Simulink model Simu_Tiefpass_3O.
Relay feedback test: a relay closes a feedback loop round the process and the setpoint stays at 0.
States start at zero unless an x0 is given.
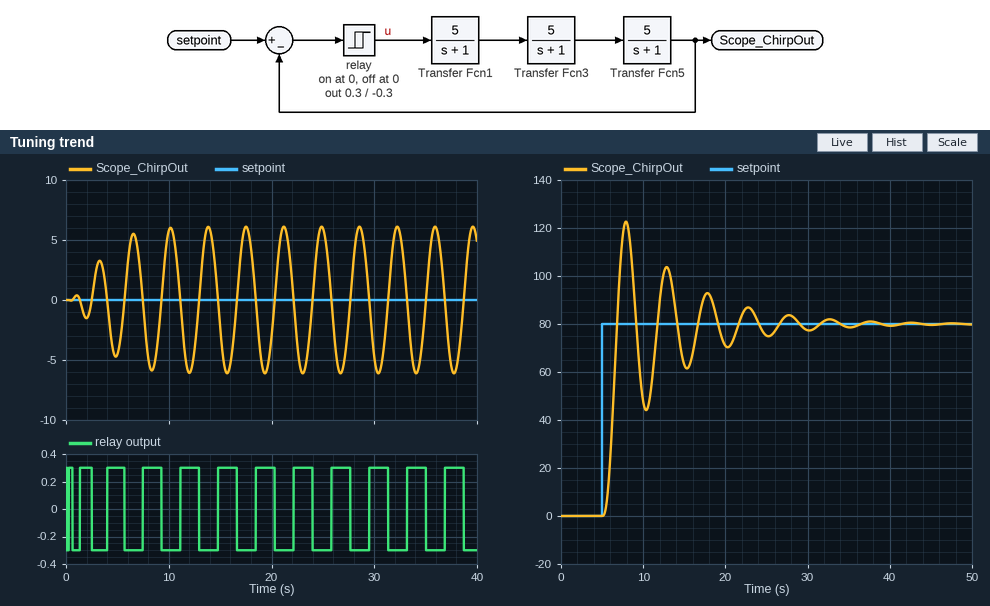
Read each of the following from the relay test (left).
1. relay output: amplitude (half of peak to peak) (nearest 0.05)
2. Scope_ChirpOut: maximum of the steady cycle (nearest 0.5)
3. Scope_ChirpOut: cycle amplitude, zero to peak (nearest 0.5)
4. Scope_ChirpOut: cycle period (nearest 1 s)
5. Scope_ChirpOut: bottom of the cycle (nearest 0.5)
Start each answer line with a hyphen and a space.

- 0.30
- 6.0
- 6.0
- 4 s
- -6.0
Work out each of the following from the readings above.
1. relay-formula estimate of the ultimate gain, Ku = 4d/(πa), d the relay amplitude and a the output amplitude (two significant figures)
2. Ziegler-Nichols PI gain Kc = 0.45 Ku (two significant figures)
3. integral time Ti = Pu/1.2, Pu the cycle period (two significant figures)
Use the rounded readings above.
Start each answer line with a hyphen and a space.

- 0.064
- 0.029
- 3.3 s
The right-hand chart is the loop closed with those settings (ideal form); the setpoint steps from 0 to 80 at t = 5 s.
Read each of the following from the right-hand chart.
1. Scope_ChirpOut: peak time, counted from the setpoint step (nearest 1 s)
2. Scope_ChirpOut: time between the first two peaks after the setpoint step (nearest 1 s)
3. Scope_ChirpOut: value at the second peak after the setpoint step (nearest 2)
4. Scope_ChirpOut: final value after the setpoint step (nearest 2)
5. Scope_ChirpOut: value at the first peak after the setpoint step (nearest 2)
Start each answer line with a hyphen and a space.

- 3 s
- 5 s
- 104
- 80
- 122
